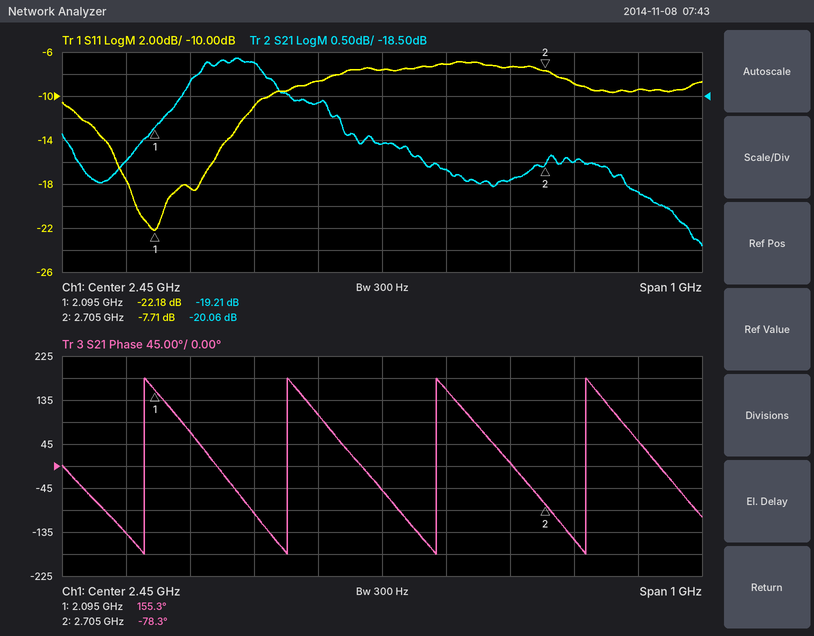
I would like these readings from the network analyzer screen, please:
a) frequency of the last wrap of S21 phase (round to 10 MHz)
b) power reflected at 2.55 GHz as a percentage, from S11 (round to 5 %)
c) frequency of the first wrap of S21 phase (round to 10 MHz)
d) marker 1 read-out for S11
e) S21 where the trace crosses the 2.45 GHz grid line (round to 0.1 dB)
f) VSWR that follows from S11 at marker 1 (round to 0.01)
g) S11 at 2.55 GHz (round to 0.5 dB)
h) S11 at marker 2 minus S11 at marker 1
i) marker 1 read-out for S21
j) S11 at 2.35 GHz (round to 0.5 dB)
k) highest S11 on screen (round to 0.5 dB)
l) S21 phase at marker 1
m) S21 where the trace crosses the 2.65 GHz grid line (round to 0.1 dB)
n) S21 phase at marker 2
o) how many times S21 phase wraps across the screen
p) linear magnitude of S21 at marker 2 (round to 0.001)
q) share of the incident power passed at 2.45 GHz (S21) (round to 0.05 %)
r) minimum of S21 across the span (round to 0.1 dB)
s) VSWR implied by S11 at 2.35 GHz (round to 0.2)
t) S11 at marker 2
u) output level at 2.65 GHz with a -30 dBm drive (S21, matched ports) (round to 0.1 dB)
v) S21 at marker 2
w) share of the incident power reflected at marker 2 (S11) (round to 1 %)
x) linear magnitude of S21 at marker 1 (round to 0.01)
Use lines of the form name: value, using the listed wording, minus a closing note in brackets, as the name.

frequency of the last wrap of S21 phase: 2.77 GHz
power reflected at 2.55 GHz as a percentage, from S11: 20 %
frequency of the first wrap of S21 phase: 2.08 GHz
marker 1 read-out for S11: -22.18 dB
S21 where the trace crosses the 2.45 GHz grid line: -19.6 dB
VSWR that follows from S11 at marker 1: 1.17
S11 at 2.55 GHz: -7.0 dB
S11 at marker 2 minus S11 at marker 1: 14.47 dB
marker 1 read-out for S21: -19.21 dB
S11 at 2.35 GHz: -8.5 dB
highest S11 on screen: -7.0 dB
S21 phase at marker 1: 155.3°
S21 where the trace crosses the 2.65 GHz grid line: -20.4 dB
S21 phase at marker 2: -78.3°
how many times S21 phase wraps across the screen: 4
linear magnitude of S21 at marker 2: 0.099
share of the incident power passed at 2.45 GHz (S21): 1.10 %
minimum of S21 across the span: -21.9 dB
VSWR implied by S11 at 2.35 GHz: 2.2
S11 at marker 2: -7.71 dB
output level at 2.65 GHz with a -30 dBm drive (S21, matched ports): -50.4 dBm
S21 at marker 2: -20.06 dB
share of the incident power reflected at marker 2 (S11): 17 %
linear magnitude of S21 at marker 1: 0.11
